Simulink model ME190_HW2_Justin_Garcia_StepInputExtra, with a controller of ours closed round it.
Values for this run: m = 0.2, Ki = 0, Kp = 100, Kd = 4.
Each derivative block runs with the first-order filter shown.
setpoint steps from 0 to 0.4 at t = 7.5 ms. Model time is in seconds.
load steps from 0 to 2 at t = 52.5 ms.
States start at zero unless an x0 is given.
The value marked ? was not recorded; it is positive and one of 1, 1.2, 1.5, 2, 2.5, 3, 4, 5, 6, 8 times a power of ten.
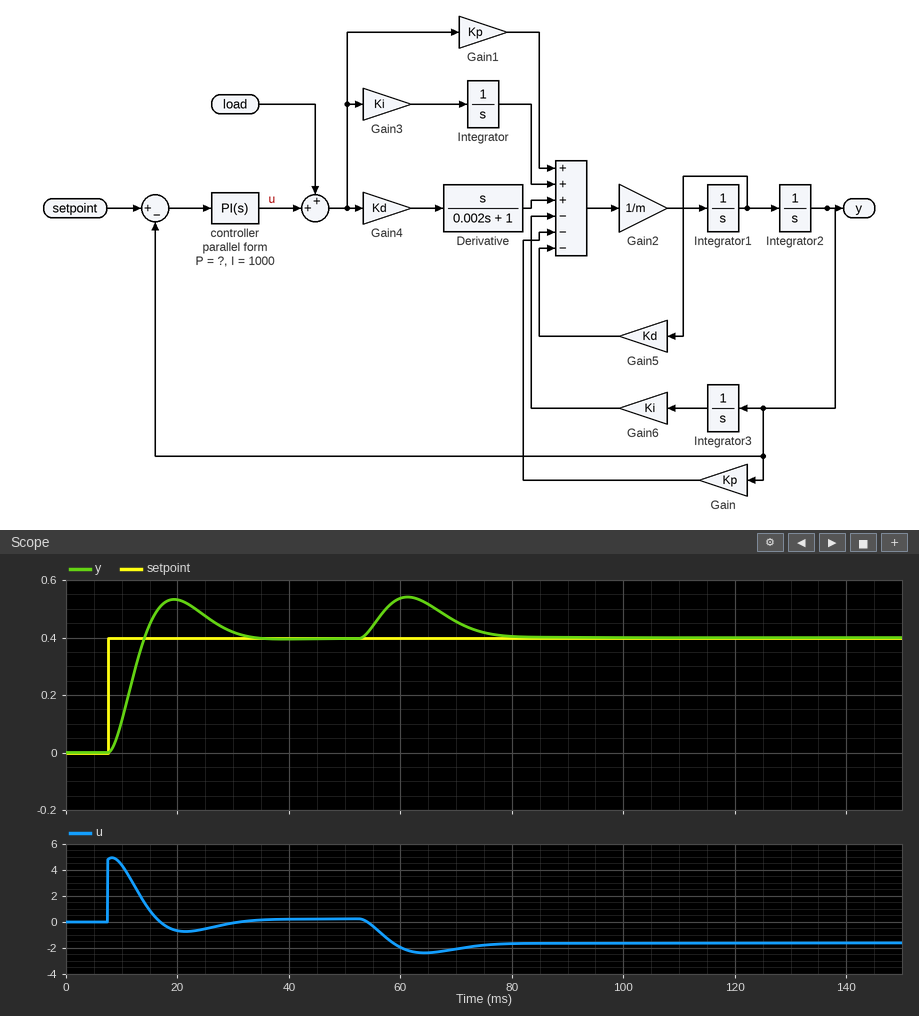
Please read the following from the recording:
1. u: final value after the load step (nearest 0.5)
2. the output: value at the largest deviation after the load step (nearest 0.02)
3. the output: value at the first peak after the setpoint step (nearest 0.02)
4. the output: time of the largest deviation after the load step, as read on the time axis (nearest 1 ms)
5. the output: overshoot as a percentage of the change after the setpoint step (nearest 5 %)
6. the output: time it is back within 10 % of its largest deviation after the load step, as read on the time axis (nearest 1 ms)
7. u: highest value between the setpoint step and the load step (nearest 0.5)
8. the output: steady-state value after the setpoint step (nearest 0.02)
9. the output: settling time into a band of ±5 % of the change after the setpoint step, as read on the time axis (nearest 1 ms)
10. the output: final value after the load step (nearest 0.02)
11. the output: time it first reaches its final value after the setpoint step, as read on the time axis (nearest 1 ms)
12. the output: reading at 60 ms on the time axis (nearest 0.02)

-1.5
0.54
0.54
61 ms
35 %
76 ms
5.0
0.40
30 ms
0.40
14 ms
0.54
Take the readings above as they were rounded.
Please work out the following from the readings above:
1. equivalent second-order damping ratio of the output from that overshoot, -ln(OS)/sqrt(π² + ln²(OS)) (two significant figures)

0.32
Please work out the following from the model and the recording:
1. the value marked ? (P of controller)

12
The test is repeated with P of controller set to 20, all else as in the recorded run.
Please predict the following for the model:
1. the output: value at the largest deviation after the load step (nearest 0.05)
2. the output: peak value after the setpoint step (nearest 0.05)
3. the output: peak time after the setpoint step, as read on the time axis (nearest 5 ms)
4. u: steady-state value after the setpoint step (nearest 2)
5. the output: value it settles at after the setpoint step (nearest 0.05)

0.50
0.50
15 ms
0
0.40
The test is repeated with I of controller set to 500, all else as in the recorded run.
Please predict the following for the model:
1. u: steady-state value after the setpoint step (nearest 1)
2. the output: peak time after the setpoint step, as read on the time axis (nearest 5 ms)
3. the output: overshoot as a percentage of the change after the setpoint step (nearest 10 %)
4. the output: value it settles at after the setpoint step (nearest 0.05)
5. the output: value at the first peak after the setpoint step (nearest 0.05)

0
20 ms
20 %
0.40
0.50
